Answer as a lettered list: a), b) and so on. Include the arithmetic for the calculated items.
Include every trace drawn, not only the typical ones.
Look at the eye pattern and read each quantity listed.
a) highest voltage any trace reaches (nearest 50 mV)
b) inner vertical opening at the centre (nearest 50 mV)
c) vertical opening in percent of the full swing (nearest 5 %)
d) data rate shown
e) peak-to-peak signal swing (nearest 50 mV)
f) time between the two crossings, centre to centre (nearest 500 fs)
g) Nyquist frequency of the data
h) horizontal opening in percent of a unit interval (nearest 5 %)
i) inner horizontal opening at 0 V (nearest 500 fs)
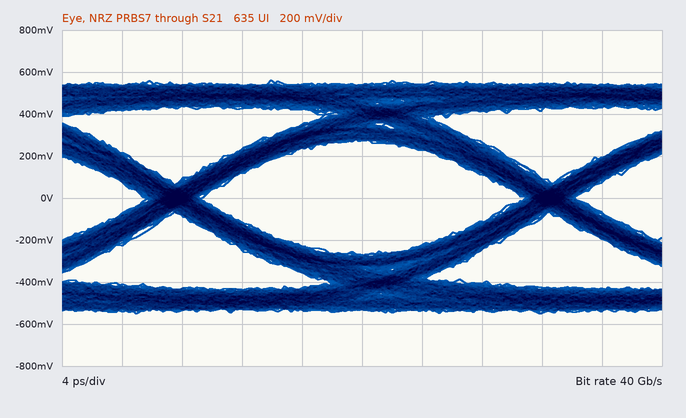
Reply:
a) 550 mV
b) 550 mV
c) 550 mV / 1.10 V ≈ 50 %
d) 40 Gb/s
e) 1.10 V
f) 25.0 ps
g) 20 GHz
h) 21.5 ps / 25.0 ps ≈ 86.0 %, so 85 % to the nearest 5 %
i) 21.5 ps
